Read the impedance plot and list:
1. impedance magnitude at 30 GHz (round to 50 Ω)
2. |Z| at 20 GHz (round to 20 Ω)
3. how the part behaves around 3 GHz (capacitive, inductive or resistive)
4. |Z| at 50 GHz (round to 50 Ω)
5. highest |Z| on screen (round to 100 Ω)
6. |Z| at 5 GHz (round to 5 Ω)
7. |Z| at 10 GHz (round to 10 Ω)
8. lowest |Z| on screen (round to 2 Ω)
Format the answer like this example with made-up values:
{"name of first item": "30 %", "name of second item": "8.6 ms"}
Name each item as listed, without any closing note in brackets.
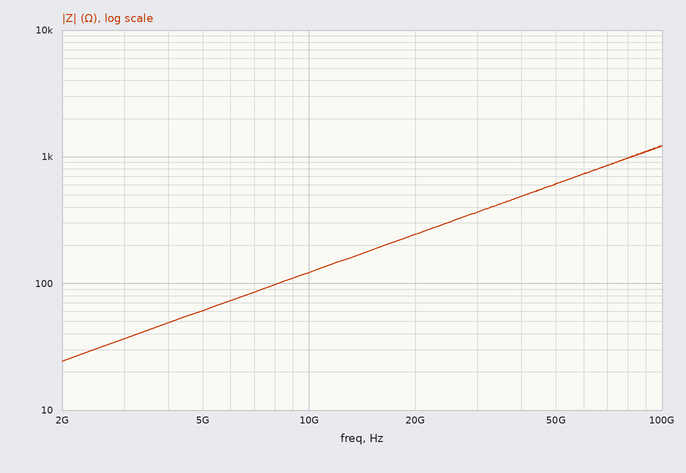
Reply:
{"impedance magnitude at 30 GHz": "350 Ω", "|Z| at 20 GHz": "240 Ω", "how the part behaves around 3 GHz": "inductive", "|Z| at 50 GHz": "600 Ω", "highest |Z| on screen": "1.2 kΩ", "|Z| at 5 GHz": "60 Ω", "|Z| at 10 GHz": "120 Ω", "lowest |Z| on screen": "24 Ω"}
